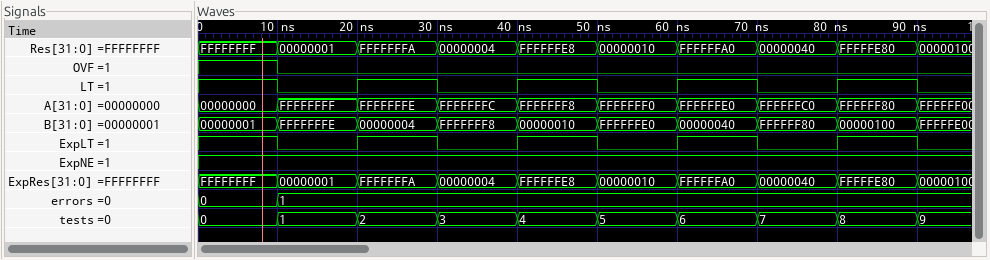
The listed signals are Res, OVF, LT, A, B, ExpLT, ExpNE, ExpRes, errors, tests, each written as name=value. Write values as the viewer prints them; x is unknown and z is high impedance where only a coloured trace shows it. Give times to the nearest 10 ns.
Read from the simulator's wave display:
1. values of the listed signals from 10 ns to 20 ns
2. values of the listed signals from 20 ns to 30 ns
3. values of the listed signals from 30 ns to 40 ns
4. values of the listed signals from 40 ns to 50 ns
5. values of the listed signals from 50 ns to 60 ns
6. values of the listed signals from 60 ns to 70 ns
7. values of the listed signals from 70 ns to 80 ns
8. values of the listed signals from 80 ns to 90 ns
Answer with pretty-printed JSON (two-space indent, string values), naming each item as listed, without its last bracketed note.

{
  "values of the listed signals from 10 ns to 20 ns": "Res=00000001, OVF=0, LT=0, A=FFFFFFFF, B=FFFFFFFE, ExpLT=0, ExpNE=1, ExpRes=00000001, errors=1, tests=1",
  "values of the listed signals from 20 ns to 30 ns": "Res=FFFFFFFA, OVF=0, LT=1, A=FFFFFFFE, B=00000004, ExpLT=1, ExpNE=1, ExpRes=FFFFFFFA, errors=1, tests=2",
  "values of the listed signals from 30 ns to 40 ns": "Res=00000004, OVF=0, LT=0, A=FFFFFFFC, B=FFFFFFF8, ExpLT=0, ExpNE=1, ExpRes=00000004, errors=1, tests=3",
  "values of the listed signals from 40 ns to 50 ns": "Res=FFFFFFE8, OVF=0, LT=1, A=FFFFFFF8, B=00000010, ExpLT=1, ExpNE=1, ExpRes=FFFFFFE8, errors=1, tests=4",
  "values of the listed signals from 50 ns to 60 ns": "Res=00000010, OVF=0, LT=0, A=FFFFFFF0, B=FFFFFFE0, ExpLT=0, ExpNE=1, ExpRes=00000010, errors=1, tests=5",
  "values of the listed signals from 60 ns to 70 ns": "Res=FFFFFFA0, OVF=0, LT=1, A=FFFFFFE0, B=00000040, ExpLT=1, ExpNE=1, ExpRes=FFFFFFA0, errors=1, tests=6",
  "values of the listed signals from 70 ns to 80 ns": "Res=00000040, OVF=0, LT=0, A=FFFFFFC0, B=FFFFFF80, ExpLT=0, ExpNE=1, ExpRes=00000040, errors=1, tests=7",
  "values of the listed signals from 80 ns to 90 ns": "Res=FFFFFE80, OVF=0, LT=1, A=FFFFFF80, B=00000100, ExpLT=1, ExpNE=1, ExpRes=FFFFFE80, errors=1, tests=8"
}
